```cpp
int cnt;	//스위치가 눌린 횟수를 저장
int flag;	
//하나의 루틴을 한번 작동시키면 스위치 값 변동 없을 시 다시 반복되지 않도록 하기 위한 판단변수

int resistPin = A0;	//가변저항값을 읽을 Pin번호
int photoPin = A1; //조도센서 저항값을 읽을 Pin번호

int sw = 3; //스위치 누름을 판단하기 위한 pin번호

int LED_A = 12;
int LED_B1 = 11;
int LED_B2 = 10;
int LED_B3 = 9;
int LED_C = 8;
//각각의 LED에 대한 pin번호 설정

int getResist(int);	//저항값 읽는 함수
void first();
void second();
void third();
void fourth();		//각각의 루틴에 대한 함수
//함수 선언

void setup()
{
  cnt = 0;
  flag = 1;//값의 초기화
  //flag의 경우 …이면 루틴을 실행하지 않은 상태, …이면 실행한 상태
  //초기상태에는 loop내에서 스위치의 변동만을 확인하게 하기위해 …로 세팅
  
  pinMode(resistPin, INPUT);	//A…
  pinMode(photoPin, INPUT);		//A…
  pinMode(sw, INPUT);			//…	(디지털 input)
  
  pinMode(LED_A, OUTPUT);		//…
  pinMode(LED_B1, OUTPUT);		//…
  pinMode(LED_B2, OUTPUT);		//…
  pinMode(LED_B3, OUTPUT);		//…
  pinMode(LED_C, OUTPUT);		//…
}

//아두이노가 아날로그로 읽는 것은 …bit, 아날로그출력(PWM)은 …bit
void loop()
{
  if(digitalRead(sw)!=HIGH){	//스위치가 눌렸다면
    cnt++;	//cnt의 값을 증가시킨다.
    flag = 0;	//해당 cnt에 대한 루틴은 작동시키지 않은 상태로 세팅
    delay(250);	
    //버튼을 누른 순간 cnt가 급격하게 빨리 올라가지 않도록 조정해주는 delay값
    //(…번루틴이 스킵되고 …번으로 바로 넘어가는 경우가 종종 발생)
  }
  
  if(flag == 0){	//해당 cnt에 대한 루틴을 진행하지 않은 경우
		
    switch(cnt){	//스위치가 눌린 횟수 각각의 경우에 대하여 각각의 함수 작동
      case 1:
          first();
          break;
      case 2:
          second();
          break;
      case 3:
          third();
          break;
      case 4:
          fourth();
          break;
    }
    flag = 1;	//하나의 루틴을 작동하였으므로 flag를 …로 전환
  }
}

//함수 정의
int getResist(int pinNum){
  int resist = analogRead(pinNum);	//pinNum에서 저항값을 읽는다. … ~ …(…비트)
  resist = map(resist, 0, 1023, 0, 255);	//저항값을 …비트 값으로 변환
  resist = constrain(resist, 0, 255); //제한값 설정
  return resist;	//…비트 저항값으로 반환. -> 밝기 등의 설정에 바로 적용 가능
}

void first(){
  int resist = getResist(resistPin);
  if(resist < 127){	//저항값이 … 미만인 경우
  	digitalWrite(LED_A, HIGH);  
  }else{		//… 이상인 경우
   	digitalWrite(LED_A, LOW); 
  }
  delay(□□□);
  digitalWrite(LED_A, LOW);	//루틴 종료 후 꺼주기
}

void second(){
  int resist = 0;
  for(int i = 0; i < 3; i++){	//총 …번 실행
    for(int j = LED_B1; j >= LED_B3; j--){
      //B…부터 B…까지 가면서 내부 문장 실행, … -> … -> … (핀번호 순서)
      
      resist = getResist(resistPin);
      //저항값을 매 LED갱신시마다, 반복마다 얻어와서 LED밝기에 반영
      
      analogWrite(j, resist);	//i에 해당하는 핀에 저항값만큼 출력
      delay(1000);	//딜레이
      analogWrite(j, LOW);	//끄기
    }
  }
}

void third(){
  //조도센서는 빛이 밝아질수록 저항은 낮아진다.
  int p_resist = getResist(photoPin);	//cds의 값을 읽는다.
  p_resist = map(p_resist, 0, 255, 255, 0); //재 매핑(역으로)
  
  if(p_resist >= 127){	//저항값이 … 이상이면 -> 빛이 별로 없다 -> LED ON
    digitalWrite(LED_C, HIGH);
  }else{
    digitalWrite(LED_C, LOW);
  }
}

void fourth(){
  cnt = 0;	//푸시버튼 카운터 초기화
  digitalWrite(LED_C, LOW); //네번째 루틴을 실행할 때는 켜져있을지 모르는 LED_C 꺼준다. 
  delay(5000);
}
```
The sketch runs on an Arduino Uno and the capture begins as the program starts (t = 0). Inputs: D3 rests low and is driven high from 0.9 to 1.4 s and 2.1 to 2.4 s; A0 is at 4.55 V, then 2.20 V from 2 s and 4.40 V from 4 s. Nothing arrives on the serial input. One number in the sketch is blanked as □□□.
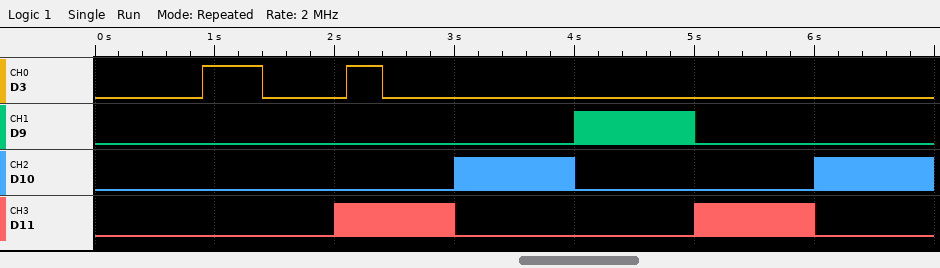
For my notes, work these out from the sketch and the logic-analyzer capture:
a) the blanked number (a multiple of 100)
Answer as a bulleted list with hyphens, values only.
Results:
- 1500
